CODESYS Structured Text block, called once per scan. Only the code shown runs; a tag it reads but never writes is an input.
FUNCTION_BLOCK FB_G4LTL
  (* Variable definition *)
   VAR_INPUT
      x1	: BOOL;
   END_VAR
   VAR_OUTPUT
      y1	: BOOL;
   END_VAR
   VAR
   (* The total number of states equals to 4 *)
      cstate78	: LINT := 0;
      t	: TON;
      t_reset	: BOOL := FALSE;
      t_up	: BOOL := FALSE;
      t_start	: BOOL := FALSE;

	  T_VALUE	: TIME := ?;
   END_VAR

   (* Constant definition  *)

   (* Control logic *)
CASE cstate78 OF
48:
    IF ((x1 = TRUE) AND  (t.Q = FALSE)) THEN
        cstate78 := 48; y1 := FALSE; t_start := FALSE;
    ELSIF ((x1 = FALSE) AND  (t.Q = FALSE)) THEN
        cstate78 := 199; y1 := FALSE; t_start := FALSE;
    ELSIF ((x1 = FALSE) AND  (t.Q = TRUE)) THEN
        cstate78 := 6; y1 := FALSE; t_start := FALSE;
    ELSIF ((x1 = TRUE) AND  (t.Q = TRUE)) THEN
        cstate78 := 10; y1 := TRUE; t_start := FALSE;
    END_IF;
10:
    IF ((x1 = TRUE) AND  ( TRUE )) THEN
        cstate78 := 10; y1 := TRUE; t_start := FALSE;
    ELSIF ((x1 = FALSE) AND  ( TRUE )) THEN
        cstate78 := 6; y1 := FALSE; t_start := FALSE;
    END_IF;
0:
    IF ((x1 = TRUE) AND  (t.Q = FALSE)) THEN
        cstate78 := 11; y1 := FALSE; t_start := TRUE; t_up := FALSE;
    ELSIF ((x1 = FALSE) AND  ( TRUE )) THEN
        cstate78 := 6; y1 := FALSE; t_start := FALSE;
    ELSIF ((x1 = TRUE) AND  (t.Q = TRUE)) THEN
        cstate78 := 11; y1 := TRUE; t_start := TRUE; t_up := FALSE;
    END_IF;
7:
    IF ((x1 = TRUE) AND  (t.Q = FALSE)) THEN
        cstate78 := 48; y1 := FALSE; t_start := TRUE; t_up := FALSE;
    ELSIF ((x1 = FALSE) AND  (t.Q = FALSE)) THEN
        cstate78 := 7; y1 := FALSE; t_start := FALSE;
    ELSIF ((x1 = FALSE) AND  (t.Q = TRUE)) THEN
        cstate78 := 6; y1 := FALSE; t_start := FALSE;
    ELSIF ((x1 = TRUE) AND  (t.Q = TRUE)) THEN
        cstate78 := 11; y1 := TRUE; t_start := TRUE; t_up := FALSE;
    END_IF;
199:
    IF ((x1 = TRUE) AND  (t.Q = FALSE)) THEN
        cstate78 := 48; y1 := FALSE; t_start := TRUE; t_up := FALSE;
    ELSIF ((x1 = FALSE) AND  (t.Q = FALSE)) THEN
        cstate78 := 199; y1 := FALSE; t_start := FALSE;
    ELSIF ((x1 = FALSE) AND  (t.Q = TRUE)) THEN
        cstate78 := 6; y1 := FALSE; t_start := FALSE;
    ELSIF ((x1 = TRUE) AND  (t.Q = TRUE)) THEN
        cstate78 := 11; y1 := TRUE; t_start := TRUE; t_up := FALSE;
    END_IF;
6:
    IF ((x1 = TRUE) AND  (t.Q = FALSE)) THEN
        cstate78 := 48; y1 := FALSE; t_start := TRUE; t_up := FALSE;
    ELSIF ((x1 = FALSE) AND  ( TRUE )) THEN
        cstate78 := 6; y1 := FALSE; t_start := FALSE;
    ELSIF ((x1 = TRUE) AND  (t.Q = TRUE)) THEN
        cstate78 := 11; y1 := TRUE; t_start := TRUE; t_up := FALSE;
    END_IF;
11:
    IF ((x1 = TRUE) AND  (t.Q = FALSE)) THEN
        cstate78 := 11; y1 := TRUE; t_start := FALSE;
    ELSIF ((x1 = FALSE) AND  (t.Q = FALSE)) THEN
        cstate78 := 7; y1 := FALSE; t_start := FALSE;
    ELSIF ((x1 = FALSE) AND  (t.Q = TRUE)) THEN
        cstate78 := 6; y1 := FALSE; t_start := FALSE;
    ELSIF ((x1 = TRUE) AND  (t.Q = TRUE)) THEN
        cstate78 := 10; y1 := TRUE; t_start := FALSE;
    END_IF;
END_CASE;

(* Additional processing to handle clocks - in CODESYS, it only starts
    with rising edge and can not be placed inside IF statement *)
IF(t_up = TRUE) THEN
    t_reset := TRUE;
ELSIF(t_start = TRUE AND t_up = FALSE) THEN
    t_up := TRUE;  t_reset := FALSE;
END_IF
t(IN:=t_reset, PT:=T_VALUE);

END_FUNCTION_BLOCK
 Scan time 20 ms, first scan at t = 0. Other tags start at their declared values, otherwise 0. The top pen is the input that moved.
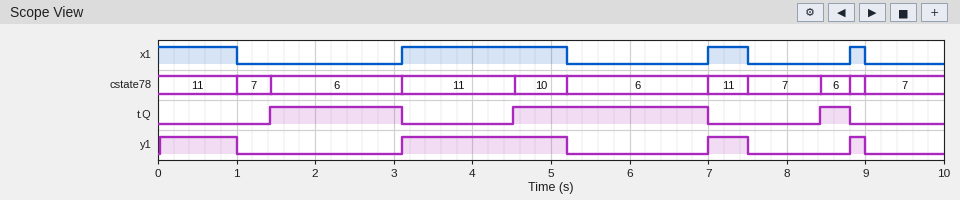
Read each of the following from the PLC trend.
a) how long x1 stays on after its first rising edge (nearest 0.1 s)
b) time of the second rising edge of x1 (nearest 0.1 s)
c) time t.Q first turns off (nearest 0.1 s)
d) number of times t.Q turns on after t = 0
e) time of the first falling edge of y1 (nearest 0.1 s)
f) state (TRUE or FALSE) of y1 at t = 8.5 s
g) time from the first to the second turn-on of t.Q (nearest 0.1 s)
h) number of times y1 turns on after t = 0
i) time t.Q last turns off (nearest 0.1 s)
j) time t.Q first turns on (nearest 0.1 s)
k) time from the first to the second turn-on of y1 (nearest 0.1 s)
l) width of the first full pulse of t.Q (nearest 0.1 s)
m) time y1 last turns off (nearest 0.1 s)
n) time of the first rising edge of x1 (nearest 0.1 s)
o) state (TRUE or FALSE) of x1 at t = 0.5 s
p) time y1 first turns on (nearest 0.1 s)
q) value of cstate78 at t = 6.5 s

2.1 s
7.0 s
3.1 s
3
1.0 s
FALSE
3.1 s
4
8.8 s
1.4 s
3.1 s
1.7 s
9.0 s
3.1 s
TRUE
0.0 s
6
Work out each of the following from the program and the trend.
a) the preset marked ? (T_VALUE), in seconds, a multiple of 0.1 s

1.4 s
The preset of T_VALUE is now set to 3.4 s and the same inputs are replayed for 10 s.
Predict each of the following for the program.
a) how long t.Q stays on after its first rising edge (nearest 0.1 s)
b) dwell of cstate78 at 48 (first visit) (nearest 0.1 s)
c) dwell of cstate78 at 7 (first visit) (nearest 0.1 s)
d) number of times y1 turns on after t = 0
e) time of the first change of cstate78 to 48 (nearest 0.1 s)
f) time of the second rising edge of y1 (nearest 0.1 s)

0.5 s
2.1 s
2.1 s
2
3.1 s
7.0 s
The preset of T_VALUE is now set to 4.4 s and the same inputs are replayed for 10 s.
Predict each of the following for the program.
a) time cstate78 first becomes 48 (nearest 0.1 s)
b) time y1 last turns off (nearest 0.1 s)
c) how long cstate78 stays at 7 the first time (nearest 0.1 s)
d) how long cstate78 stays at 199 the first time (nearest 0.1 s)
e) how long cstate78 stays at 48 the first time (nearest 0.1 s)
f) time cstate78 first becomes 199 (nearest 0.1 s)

3.1 s
1.0 s
2.1 s
1.8 s
2.1 s
5.2 s
